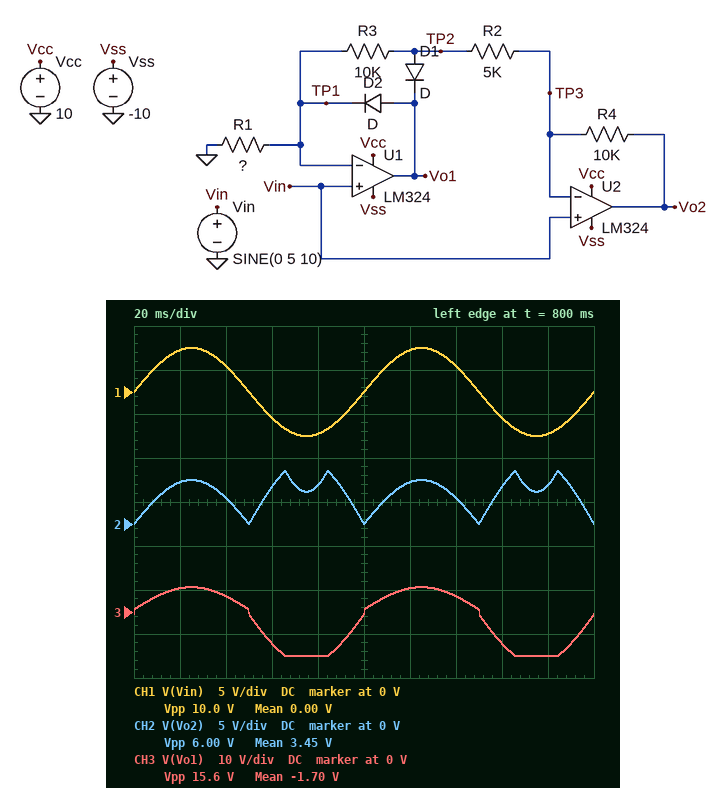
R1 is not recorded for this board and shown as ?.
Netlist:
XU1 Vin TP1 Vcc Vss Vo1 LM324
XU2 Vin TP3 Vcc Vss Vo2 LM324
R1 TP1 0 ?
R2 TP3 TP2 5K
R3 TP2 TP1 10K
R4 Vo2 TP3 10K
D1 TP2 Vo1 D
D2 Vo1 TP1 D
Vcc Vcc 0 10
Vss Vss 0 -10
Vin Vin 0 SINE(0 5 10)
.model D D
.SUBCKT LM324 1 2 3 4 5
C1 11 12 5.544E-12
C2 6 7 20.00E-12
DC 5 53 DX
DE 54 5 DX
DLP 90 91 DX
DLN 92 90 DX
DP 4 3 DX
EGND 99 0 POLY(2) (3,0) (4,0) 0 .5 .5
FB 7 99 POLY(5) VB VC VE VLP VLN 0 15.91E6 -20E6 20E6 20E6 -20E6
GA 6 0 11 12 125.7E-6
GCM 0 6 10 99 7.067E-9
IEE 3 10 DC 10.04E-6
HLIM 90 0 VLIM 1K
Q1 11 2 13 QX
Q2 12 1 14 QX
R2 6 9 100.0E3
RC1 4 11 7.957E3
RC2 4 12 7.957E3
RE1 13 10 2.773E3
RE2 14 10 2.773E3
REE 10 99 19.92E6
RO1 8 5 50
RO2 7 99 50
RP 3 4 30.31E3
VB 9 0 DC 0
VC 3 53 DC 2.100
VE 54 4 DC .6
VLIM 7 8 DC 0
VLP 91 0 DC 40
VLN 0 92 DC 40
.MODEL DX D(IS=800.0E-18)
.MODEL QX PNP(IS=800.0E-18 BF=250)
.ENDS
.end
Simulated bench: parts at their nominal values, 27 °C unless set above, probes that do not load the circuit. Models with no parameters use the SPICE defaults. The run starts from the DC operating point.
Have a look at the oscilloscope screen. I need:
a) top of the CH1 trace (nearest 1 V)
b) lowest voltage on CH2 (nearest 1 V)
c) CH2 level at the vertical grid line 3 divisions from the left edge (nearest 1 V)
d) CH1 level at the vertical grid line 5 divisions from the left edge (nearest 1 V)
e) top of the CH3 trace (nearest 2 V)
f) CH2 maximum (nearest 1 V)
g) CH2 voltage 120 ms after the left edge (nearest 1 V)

5 V
0 V
4 V
0 V
6 V
6 V
5 V
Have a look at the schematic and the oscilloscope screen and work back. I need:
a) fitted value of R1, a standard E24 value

8.2 kΩ
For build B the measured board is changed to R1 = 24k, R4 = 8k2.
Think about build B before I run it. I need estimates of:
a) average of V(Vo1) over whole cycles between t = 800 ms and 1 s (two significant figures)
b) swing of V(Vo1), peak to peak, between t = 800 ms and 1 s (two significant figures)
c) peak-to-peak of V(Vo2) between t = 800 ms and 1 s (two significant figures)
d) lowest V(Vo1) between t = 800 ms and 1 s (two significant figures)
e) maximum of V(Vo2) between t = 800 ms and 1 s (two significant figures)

-680 mV
13 V
6.6 V
-7.7 V
5.0 V
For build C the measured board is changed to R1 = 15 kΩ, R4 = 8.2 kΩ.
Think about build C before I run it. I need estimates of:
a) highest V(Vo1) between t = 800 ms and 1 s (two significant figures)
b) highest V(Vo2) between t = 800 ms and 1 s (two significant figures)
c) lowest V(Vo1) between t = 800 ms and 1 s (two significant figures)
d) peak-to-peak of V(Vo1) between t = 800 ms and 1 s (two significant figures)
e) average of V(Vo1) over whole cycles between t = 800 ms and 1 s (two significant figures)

5.6 V
5.0 V
-9.0 V
15 V
-1.1 V
